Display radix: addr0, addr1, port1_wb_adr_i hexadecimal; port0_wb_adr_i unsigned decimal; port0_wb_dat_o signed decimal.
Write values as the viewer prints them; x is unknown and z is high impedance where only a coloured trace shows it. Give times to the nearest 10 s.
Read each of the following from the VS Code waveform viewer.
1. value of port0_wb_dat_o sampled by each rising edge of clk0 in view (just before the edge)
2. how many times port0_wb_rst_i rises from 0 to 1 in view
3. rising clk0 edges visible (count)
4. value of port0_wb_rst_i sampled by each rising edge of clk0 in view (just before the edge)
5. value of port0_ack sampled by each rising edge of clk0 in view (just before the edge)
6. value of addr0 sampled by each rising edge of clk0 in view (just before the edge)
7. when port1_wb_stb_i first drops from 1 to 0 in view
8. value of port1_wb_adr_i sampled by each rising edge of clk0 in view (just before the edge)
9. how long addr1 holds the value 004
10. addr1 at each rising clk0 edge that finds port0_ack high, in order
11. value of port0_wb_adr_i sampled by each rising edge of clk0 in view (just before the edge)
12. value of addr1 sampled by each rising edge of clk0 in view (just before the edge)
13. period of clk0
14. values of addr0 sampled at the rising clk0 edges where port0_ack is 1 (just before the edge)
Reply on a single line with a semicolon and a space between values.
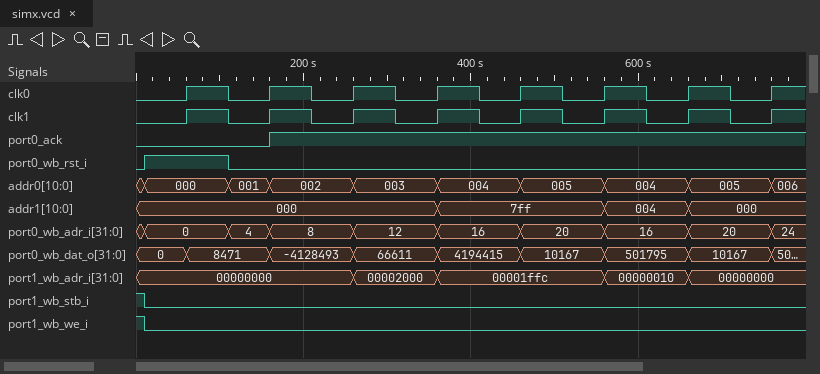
0, 8471, -4128493, 66611, 4194415, 10167, 501795, 10167; 1; 8; 1 0 0 0 0 0 0 0; 0 0 1 1 1 1 1 1; 000, 001, 002, 003, 004, 005, 004, 005; 10 s; 00000000, 00000000, 00000000, 00002000, 00001ffc, 00001ffc, 00000010, 00000000; 100 s; 000, 000, 7ff, 7ff, 004, 000; 0, 4, 8, 12, 16, 20, 16, 20; 000, 000, 000, 000, 7ff, 7ff, 004, 000; 100 s; 002, 003, 004, 005, 004, 005
